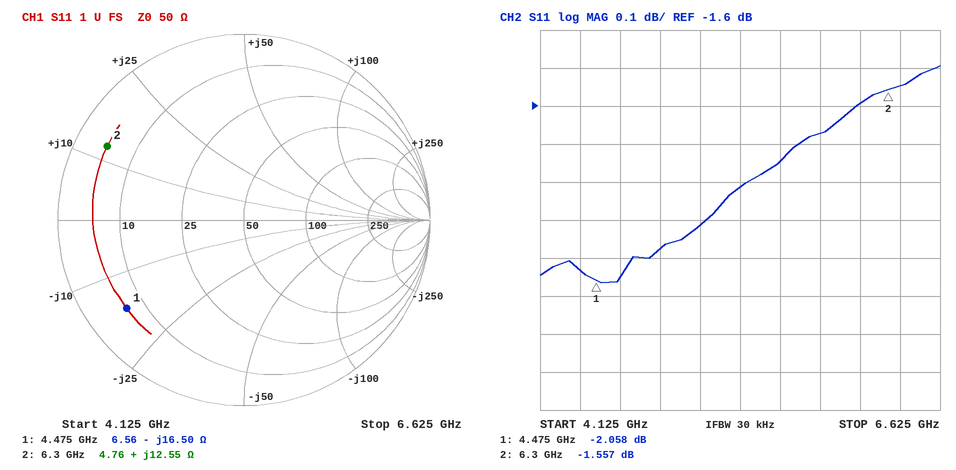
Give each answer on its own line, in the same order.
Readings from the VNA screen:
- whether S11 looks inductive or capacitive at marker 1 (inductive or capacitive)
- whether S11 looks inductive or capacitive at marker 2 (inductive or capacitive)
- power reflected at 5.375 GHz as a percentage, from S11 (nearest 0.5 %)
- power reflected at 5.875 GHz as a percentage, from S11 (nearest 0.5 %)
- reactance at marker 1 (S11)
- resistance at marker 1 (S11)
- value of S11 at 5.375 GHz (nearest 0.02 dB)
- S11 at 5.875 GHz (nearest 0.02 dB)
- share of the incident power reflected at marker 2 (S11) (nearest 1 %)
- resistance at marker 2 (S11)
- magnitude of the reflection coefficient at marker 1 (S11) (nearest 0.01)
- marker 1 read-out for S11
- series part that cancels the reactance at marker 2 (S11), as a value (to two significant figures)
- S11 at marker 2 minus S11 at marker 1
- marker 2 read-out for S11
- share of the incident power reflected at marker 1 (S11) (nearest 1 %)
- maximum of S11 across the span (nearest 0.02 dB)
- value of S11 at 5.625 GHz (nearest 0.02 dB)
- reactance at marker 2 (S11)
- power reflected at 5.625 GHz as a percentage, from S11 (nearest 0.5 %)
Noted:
capacitive
inductive
66.0 %
68.0 %
-16.50 Ω
6.56 Ω
-1.82 dB
-1.68 dB
70 %
4.76 Ω
0.79
-2.058 dB
2.0 pF
0.501 dB
-1.557 dB
62 %
-1.50 dB
-1.74 dB
+12.55 Ω
67.0 %
